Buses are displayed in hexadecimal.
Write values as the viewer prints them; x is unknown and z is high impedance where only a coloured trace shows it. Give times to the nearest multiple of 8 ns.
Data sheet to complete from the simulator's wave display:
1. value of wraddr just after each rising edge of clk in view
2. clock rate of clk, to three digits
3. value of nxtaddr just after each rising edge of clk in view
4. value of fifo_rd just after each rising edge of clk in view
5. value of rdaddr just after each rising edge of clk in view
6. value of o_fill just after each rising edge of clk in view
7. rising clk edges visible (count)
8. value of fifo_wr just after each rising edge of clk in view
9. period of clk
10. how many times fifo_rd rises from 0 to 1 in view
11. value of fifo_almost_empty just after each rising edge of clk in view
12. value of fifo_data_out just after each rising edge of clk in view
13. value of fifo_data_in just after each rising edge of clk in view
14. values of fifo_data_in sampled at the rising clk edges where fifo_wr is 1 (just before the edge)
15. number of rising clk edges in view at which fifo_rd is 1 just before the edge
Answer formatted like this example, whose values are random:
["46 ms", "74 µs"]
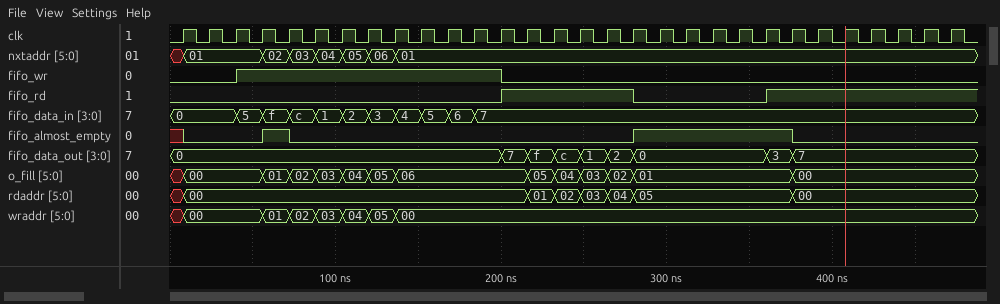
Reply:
["00, 00, 00, 01, 02, 03, 04, 05, 00, 00, 00, 00, 00, 00, 00, 00, 00, 00, 00, 00, 00, 00, 00, 00, 00, 00, 00, 00, 00, 00", "62.5 MHz", "01, 01, 01, 02, 03, 04, 05, 06, 01, 01, 01, 01, 01, 01, 01, 01, 01, 01, 01, 01, 01, 01, 01, 01, 01, 01, 01, 01, 01, 01", "0 0 0 0 0 0 0 0 0 0 0 0 1 1 1 1 1 0 0 0 0 0 1 1 1 1 1 1 1 1", "00, 00, 00, 00, 00, 00, 00, 00, 00, 00, 00, 00, 00, 01, 02, 03, 04, 05, 05, 05, 05, 05, 05, 00, 00, 00, 00, 00, 00, 00", "00, 00, 00, 01, 02, 03, 04, 05, 06, 06, 06, 06, 06, 05, 04, 03, 02, 01, 01, 01, 01, 01, 01, 00, 00, 00, 00, 00, 00, 00", "30", "0 0 1 1 1 1 1 1 1 1 1 1 0 0 0 0 0 0 0 0 0 0 0 0 0 0 0 0 0 0", "16 ns", "2", "0 0 0 1 0 0 0 0 0 0 0 0 0 0 0 0 0 1 1 1 1 1 1 0 0 0 0 0 0 0", "0, 0, 0, 0, 0, 0, 0, 0, 0, 0, 0, 0, 7, f, c, 1, 2, 0, 0, 0, 0, 0, 3, 7, 7, 7, 7, 7, 7, 7", "0, 0, 5, f, c, 1, 2, 3, 4, 5, 6, 7, 7, 7, 7, 7, 7, 7, 7, 7, 7, 7, 7, 7, 7, 7, 7, 7, 7, 7", "5, f, c, 1, 2, 3, 4, 5, 6, 7", "12"]
